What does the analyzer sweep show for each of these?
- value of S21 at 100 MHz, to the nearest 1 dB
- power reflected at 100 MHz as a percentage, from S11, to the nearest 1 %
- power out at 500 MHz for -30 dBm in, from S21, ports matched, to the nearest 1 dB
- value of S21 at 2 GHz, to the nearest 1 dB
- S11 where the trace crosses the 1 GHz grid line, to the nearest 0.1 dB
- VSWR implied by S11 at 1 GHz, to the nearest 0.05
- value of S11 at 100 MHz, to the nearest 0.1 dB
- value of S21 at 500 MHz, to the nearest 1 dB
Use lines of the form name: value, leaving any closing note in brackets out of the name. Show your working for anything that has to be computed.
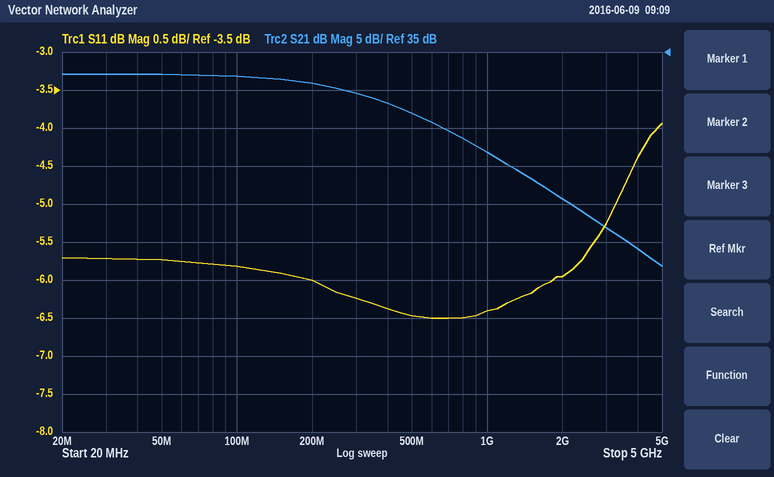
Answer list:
value of S21 at 100 MHz, to the nearest 1 dB: 32 dB
power reflected at 100 MHz as a percentage, from S11, to the nearest 1 %: 10^(-5.8/10) ≈ 26 %
power out at 500 MHz for -30 dBm in, from S21, ports matched, to the nearest 1 dB: -30 dBm + (27 dB) = -3 dBm
value of S21 at 2 GHz, to the nearest 1 dB: 16 dB
S11 where the trace crosses the 1 GHz grid line, to the nearest 0.1 dB: -6.4 dB
VSWR implied by S11 at 1 GHz, to the nearest 0.05: |Γ| = 10^(-6.4/20) = 0.4786; VSWR = (1 + 0.4786)/(1 − 0.4786) ≈ 2.84, so 2.85 to the nearest 0.05
value of S11 at 100 MHz, to the nearest 0.1 dB: -5.8 dB
value of S21 at 500 MHz, to the nearest 1 dB: 27 dB
